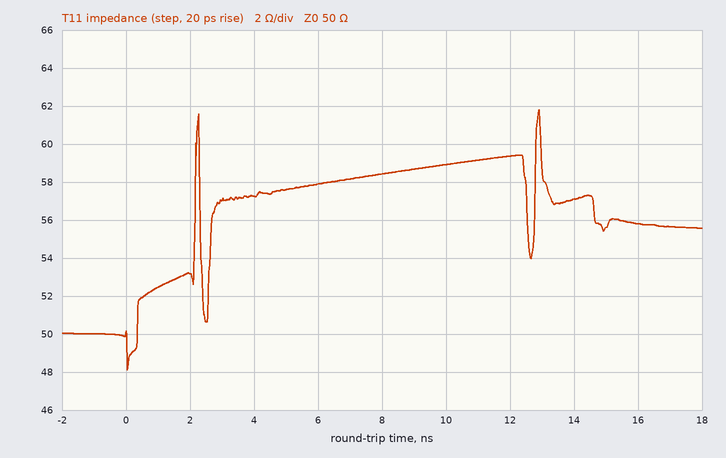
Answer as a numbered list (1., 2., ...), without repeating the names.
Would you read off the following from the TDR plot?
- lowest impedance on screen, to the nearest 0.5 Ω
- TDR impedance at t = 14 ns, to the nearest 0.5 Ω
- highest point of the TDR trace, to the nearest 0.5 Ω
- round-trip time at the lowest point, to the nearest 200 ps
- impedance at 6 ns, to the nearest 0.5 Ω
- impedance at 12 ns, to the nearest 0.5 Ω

1. 48.0 Ω
2. 57.0 Ω
3. 62.0 Ω
4. 0.0 ns
5. 58.0 Ω
6. 59.5 Ω
